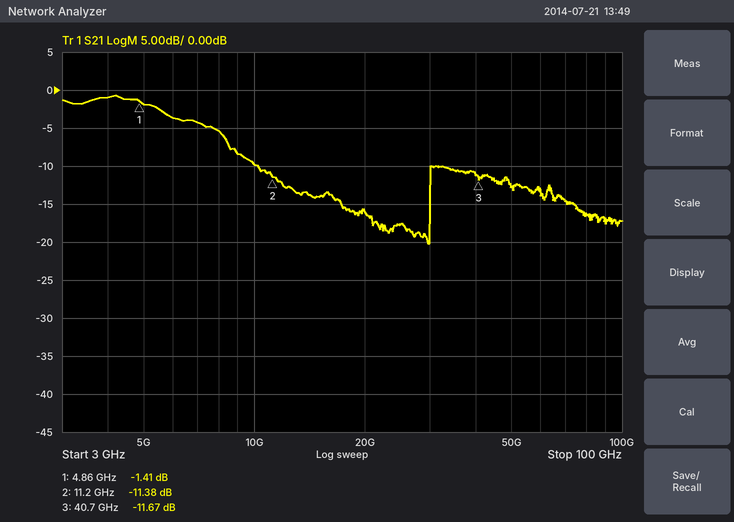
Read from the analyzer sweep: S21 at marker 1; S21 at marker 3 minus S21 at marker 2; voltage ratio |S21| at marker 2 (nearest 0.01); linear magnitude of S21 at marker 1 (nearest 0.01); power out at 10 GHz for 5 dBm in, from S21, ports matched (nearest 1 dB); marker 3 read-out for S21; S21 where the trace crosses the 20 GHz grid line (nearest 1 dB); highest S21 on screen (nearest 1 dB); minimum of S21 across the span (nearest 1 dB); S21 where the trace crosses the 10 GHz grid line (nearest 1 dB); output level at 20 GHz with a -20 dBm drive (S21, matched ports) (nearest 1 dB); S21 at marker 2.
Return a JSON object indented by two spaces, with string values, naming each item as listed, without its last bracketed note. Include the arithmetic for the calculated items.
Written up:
{
  "S21 at marker 1": "-1.41 dB",
  "S21 at marker 3 minus S21 at marker 2": "-11.67 − (-11.38) = -0.29 dB",
  "voltage ratio |S21| at marker 2": "10^(-11.38/20) ≈ 0.27",
  "linear magnitude of S21 at marker 1": "10^(-1.41/20) ≈ 0.85",
  "power out at 10 GHz for 5 dBm in, from S21, ports matched": "5 dBm + (-10 dB) = -5 dBm",
  "marker 3 read-out for S21": "-11.67 dB",
  "S21 where the trace crosses the 20 GHz grid line": "-16 dB",
  "highest S21 on screen": "-1 dB",
  "minimum of S21 across the span": "-20 dB",
  "S21 where the trace crosses the 10 GHz grid line": "-10 dB",
  "output level at 20 GHz with a -20 dBm drive (S21, matched ports)": "-20 dBm + (-16 dB) = -36 dBm",
  "S21 at marker 2": "-11.38 dB"
}
